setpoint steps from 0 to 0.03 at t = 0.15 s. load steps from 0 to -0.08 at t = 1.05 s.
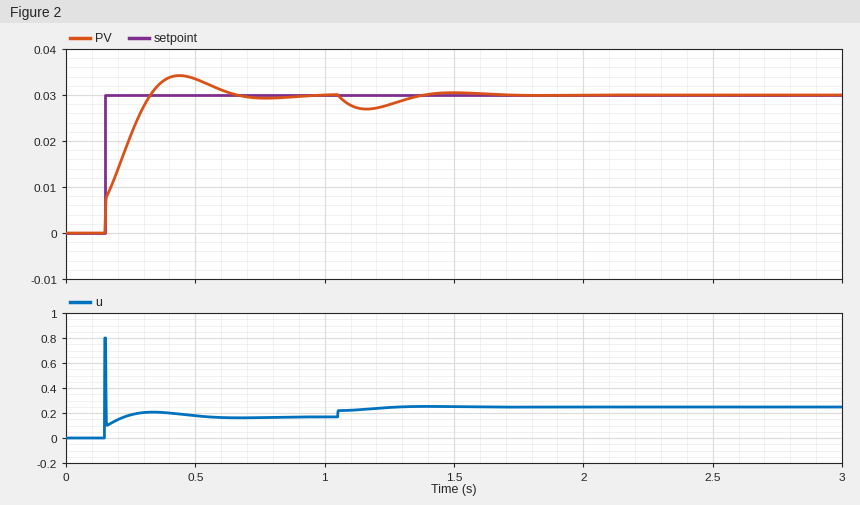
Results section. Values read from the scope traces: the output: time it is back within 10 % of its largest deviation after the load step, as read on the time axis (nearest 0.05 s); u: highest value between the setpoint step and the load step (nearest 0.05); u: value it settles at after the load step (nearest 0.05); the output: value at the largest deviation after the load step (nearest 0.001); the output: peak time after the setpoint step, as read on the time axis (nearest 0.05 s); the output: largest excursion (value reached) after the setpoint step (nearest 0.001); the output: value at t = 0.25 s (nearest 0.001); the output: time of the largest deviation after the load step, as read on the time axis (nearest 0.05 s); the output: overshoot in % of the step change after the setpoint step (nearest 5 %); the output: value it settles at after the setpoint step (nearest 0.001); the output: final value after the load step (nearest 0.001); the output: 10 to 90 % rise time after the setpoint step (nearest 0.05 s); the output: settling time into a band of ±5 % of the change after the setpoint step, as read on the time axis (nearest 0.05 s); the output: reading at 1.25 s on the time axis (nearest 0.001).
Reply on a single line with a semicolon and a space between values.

1.60 s; 0.80; 0.25; 0.027; 0.45 s; 0.034; 0.021; 1.15 s; 15 %; 0.030; 0.030; 0.15 s; 0.60 s; 0.028
